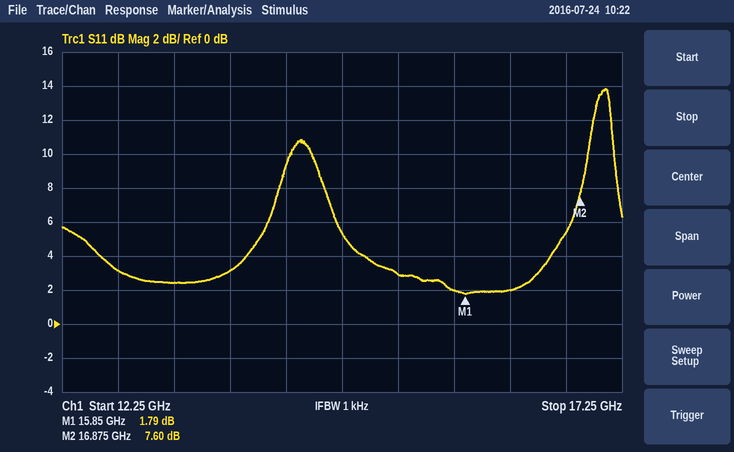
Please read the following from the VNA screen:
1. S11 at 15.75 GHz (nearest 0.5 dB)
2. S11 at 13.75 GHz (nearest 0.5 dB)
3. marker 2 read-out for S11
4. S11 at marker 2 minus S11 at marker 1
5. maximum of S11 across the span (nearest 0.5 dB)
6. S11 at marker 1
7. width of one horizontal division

2.0 dB
3.0 dB
7.60 dB
5.81 dB
14.0 dB
1.79 dB
500 MHz
